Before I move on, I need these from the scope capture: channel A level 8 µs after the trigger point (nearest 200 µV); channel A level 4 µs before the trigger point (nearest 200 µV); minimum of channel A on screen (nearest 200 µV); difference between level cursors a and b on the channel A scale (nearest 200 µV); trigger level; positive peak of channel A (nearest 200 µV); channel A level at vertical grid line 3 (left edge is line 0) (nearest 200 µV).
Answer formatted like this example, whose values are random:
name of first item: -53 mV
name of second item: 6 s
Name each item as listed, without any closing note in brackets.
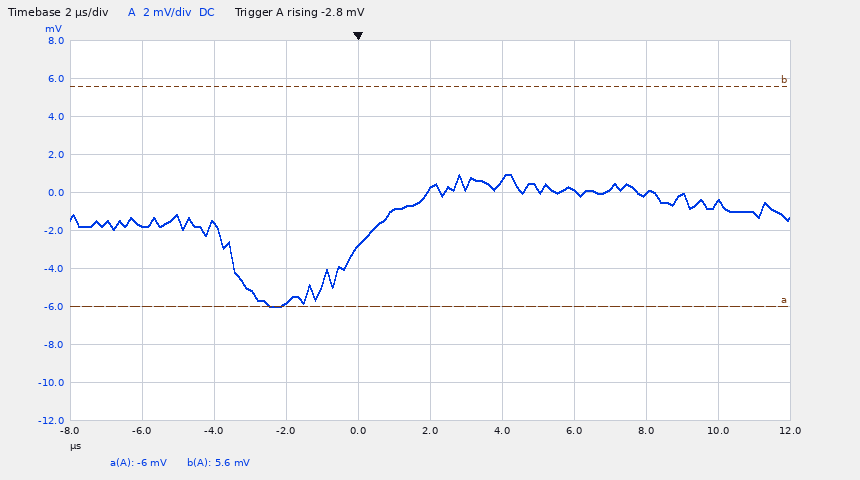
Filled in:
channel A level 8 µs after the trigger point: 0.0 mV
channel A level 4 µs before the trigger point: -1.6 mV
minimum of channel A on screen: -6.0 mV
difference between level cursors a and b on the channel A scale: 11.6 mV
trigger level: -2.8 mV
positive peak of channel A: 1.0 mV
channel A level at vertical grid line 3 (left edge is line 0): -5.8 mV
